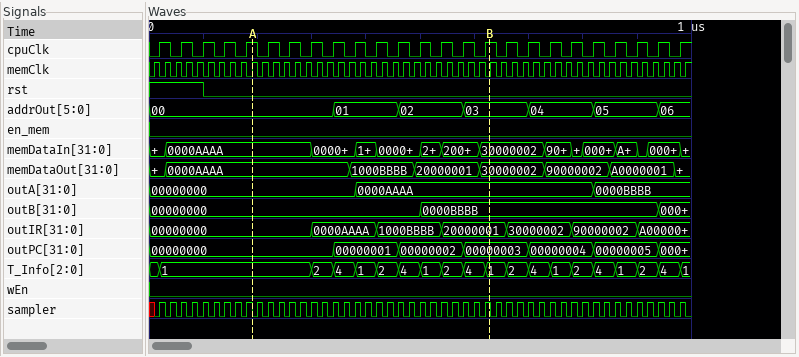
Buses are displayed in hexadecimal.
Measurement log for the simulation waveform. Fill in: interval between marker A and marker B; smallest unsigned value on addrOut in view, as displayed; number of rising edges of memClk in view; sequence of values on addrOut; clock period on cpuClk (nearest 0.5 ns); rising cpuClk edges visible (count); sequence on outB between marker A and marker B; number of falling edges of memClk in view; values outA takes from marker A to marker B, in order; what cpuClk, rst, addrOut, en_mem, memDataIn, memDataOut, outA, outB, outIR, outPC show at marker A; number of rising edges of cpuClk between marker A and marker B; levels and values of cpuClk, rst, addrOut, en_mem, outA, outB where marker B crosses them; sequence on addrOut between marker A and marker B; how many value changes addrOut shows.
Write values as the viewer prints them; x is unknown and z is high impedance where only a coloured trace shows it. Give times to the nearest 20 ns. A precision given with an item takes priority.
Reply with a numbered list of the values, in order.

1. 440 ns
2. 00
3. 50
4. 00, 01, 02, 03, 04, 05, 06
5. 40 ns
6. 25
7. 00000000, 0000BBBB
8. 49
9. 00000000, 0000AAAA
10. cpuClk=1, rst=0, addrOut=00, en_mem=0, memDataIn=0000AAAA, memDataOut=0000AAAA, outA=00000000, outB=00000000, outIR=00000000, outPC=00000000
11. 11
12. cpuClk=1, rst=0, addrOut=03, en_mem=0, outA=0000AAAA, outB=0000BBBB
13. 00, 01, 02, 03
14. 6
